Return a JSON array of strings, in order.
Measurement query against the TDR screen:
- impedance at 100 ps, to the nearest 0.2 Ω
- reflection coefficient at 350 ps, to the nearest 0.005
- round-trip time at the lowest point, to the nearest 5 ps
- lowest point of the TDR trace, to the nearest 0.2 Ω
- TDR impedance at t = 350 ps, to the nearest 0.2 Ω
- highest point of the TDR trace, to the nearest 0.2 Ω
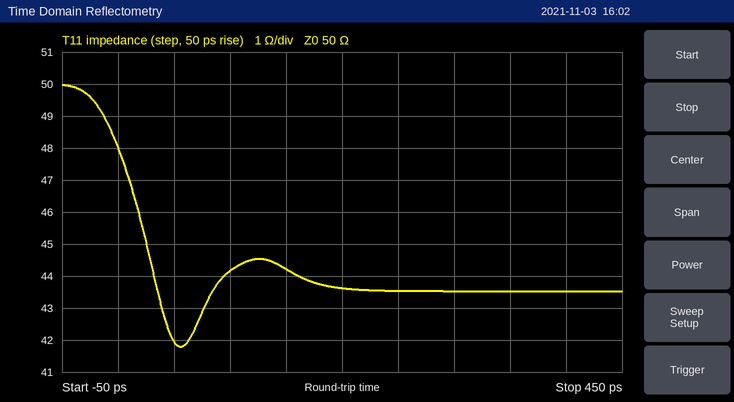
["44.2 Ω", "-0.070", "55 ps", "41.8 Ω", "43.6 Ω", "50.0 Ω"]
